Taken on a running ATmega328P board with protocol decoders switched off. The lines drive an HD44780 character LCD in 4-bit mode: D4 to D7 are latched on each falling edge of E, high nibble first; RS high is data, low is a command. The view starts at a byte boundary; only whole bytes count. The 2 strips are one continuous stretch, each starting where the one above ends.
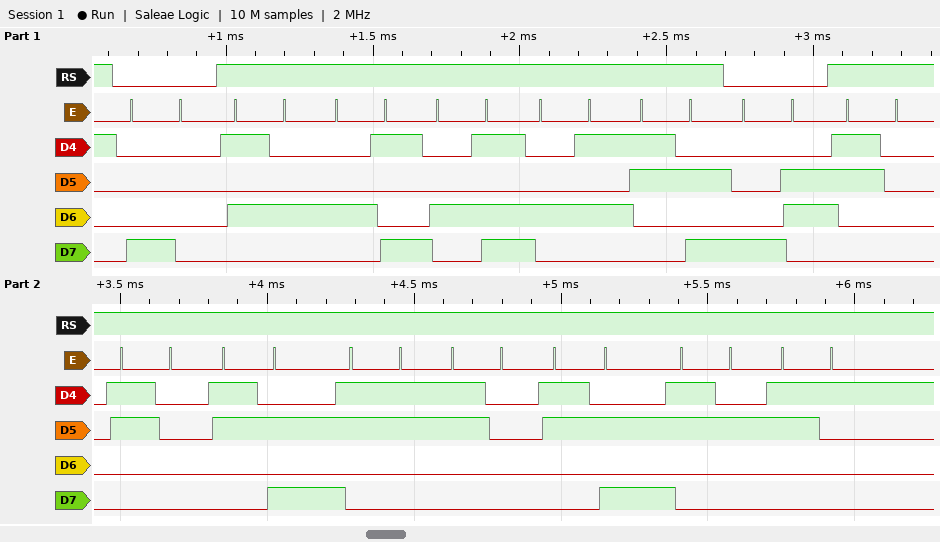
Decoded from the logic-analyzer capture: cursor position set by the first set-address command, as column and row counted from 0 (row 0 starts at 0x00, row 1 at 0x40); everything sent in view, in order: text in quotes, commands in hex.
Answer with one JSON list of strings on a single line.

["column 0, row 0", "0x80 \"TIME:\" 0x86 \"00:30:21\""]
